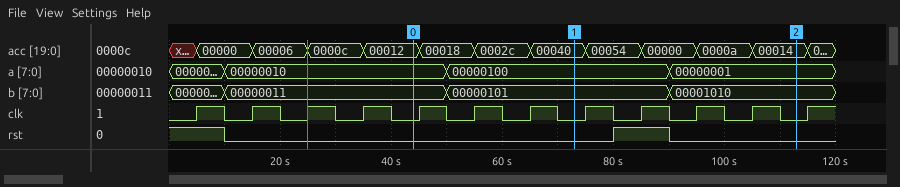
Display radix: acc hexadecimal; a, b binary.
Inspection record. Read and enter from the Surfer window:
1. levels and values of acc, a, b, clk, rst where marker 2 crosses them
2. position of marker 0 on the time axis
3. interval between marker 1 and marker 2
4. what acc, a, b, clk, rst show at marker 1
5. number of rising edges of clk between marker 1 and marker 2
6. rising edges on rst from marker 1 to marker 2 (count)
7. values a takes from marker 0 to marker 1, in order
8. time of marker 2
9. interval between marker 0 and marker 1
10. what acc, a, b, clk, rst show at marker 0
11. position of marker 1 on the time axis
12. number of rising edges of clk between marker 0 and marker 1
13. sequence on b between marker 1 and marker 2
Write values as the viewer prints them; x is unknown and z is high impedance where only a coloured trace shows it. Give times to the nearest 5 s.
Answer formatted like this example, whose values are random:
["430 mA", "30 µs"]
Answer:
["acc=00014, a=00000001, b=00001010, clk=0, rst=0", "45 s", "40 s", "acc=00040, a=00000100, b=00000101, clk=0, rst=0", "4", "1", "00000010, 00000100", "115 s", "30 s", "acc=00012, a=00000010, b=00000011, clk=0, rst=0", "75 s", "3", "00000101, 00001010"]
